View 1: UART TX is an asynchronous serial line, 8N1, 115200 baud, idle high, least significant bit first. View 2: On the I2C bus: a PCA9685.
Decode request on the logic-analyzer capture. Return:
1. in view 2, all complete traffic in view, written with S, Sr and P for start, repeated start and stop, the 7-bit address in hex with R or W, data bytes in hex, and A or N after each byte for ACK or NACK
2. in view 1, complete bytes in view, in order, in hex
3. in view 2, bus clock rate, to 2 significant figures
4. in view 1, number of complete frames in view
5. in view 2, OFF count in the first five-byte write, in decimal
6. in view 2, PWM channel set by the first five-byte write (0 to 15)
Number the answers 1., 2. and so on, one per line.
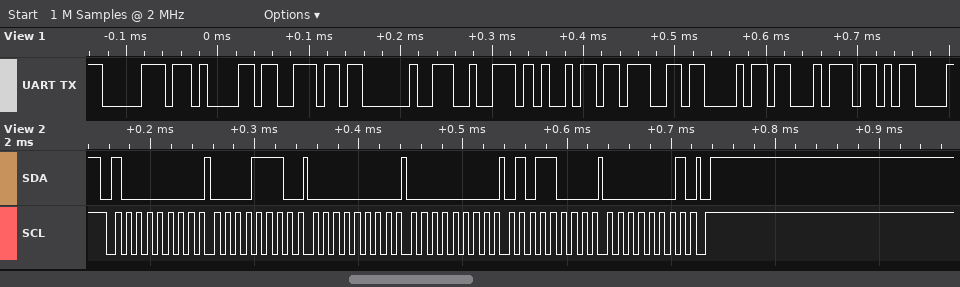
1. S 40W A 0E A 00 A 00 A 58 A 01 A P
2. 0x70 0x61 0x6E 0x20 0x72 0x69 0x67 0x68 0x74 0x0D
3. 100 kHz
4. 10
5. 344
6. 2
